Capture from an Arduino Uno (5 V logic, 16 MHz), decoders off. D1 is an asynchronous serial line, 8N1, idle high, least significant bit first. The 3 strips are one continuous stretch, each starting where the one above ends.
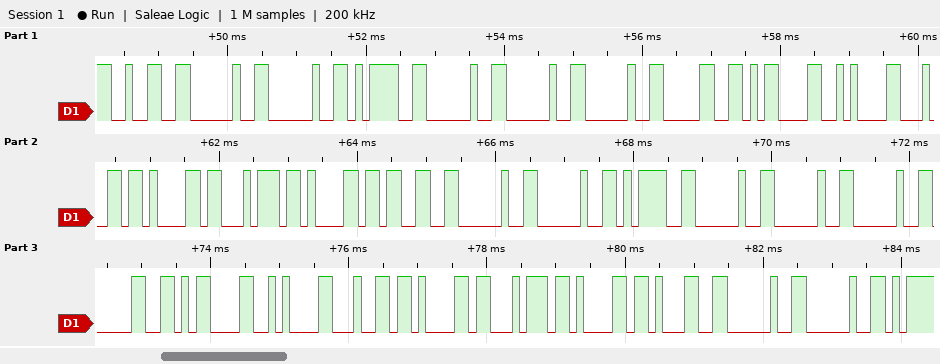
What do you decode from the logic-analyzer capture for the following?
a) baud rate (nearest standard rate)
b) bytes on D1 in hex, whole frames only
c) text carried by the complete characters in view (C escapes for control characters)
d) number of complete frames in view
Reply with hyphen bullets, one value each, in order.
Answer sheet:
- 9600 baud
- 32 20 20 3D 20 20 20 30 0D 0A 64 61 74 61 33 20 20 3D 20 20 20 30 0D 0A 64 61 74 61 31 20 20
- "2  =   0\r\ndata3  =   0\r\ndata1  "
- 31
